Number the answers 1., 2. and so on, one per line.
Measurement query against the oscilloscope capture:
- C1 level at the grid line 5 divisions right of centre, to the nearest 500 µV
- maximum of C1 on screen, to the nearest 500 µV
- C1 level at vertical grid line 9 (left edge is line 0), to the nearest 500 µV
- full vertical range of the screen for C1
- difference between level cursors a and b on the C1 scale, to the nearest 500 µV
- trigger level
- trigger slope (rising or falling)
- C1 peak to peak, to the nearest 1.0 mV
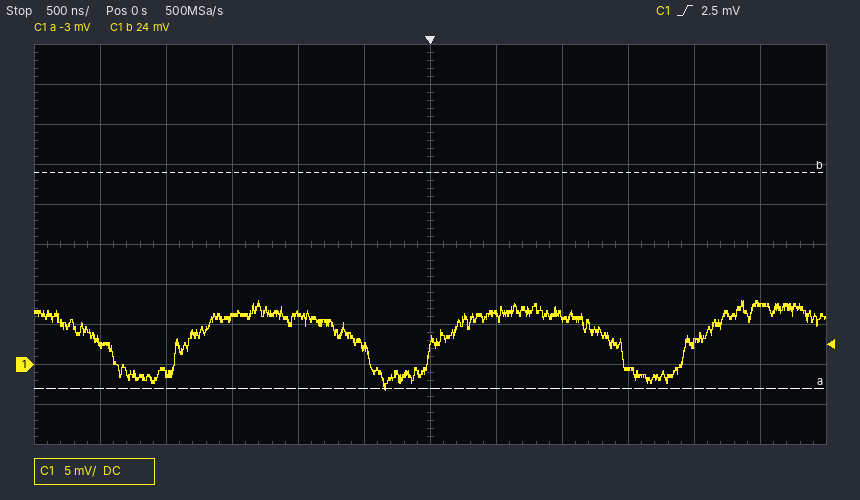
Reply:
1. 7.5 mV
2. 8.0 mV
3. -500 µV
4. 50 mV
5. 27.0 mV
6. 2.5 mV
7. rising
8. 11.0 mV
